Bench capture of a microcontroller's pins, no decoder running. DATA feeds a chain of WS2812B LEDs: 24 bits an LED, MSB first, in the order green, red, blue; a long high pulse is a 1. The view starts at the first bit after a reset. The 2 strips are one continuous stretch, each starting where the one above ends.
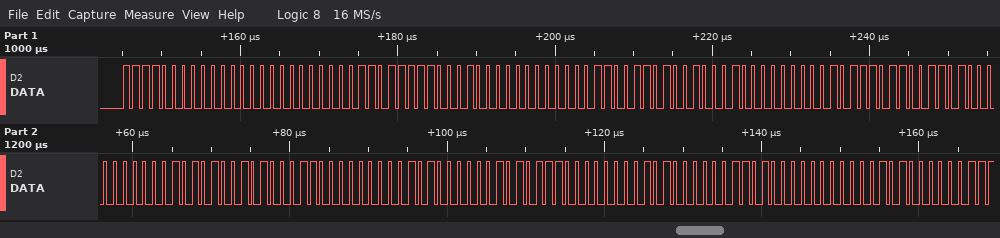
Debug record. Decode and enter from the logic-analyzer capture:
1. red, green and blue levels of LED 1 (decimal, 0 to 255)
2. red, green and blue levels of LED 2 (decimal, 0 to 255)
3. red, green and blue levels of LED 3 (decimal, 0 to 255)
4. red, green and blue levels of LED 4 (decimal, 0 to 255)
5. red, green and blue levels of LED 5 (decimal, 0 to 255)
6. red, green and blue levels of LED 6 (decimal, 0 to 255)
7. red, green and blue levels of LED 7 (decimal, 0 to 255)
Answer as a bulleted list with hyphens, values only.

- 0, 240, 0
- 16, 223, 0
- 34, 205, 0
- 52, 187, 0
- 70, 169, 0
- 87, 160, 0
- 104, 160, 0
